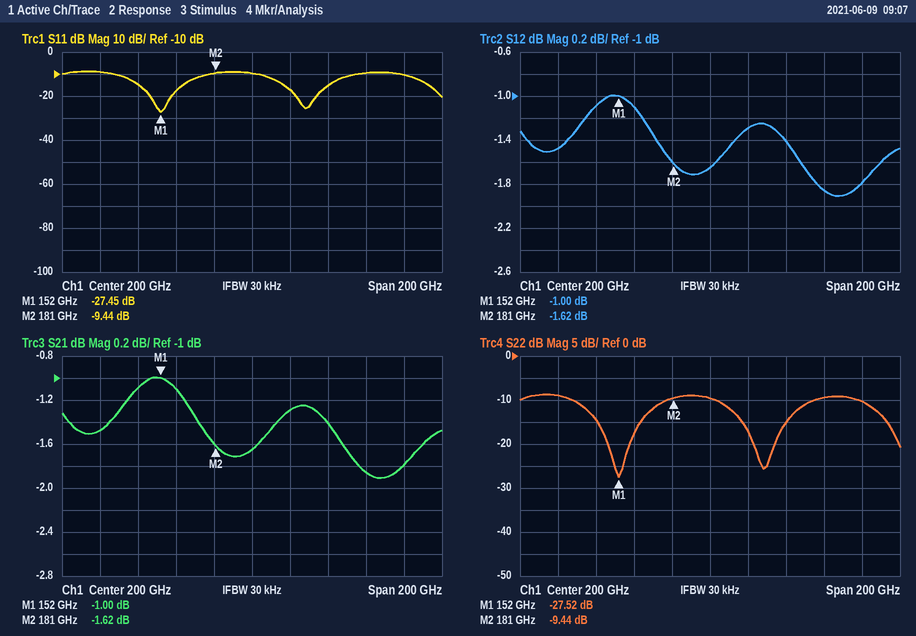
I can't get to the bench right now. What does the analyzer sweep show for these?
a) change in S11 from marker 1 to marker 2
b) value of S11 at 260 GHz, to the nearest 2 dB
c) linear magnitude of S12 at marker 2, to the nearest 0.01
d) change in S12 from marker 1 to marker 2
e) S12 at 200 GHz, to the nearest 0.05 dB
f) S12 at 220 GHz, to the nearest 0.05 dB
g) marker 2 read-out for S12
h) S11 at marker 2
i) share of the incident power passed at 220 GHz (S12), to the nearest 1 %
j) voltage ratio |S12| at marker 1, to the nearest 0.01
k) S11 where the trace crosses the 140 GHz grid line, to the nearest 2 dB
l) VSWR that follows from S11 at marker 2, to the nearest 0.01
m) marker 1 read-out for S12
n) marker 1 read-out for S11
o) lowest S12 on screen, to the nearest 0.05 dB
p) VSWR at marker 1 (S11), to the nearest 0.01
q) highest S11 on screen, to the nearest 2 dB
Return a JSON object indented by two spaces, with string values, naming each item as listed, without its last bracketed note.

{
  "change in S11 from marker 1 to marker 2": "18.01 dB",
  "value of S11 at 260 GHz, to the nearest 2 dB": "-10 dB",
  "linear magnitude of S12 at marker 2, to the nearest 0.01": "0.83",
  "change in S12 from marker 1 to marker 2": "-0.62 dB",
  "S12 at 200 GHz, to the nearest 0.05 dB": "-1.65 dB",
  "S12 at 220 GHz, to the nearest 0.05 dB": "-1.30 dB",
  "marker 2 read-out for S12": "-1.62 dB",
  "S11 at marker 2": "-9.44 dB",
  "share of the incident power passed at 220 GHz (S12), to the nearest 1 %": "74 %",
  "voltage ratio |S12| at marker 1, to the nearest 0.01": "0.89",
  "S11 where the trace crosses the 140 GHz grid line, to the nearest 2 dB": "-14 dB",
  "VSWR that follows from S11 at marker 2, to the nearest 0.01": "2.02",
  "marker 1 read-out for S12": "-1.00 dB",
  "marker 1 read-out for S11": "-27.45 dB",
  "lowest S12 on screen, to the nearest 0.05 dB": "-1.90 dB",
  "VSWR at marker 1 (S11), to the nearest 0.01": "1.09",
  "highest S11 on screen, to the nearest 2 dB": "-8 dB"
}
